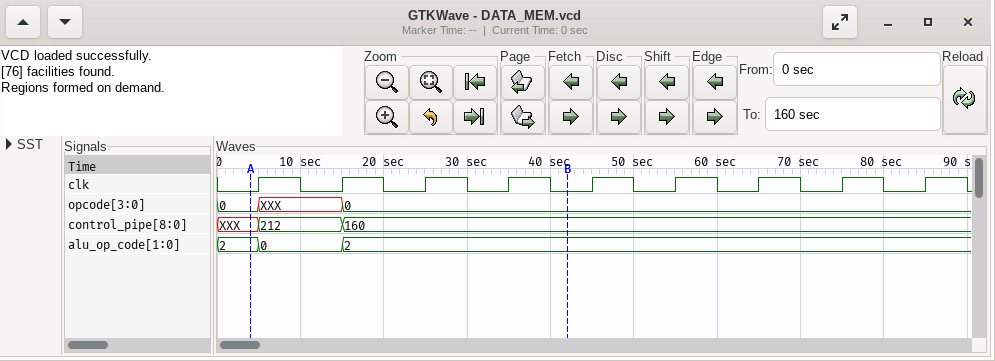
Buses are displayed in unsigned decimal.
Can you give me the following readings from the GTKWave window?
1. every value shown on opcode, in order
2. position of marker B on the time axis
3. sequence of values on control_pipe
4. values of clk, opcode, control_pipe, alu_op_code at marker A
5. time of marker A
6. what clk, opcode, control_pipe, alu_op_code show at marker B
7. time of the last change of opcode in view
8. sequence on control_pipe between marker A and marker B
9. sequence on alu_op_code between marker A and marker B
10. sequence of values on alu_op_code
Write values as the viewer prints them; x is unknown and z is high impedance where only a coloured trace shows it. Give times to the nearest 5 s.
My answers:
0, XXX, 0
40 s
XXX, 212, 160
clk=0, opcode=0, control_pipe=XXX, alu_op_code=2
5 s
clk=0, opcode=0, control_pipe=160, alu_op_code=2
15 s
XXX, 212, 160
2, 0, 2
2, 0, 2
